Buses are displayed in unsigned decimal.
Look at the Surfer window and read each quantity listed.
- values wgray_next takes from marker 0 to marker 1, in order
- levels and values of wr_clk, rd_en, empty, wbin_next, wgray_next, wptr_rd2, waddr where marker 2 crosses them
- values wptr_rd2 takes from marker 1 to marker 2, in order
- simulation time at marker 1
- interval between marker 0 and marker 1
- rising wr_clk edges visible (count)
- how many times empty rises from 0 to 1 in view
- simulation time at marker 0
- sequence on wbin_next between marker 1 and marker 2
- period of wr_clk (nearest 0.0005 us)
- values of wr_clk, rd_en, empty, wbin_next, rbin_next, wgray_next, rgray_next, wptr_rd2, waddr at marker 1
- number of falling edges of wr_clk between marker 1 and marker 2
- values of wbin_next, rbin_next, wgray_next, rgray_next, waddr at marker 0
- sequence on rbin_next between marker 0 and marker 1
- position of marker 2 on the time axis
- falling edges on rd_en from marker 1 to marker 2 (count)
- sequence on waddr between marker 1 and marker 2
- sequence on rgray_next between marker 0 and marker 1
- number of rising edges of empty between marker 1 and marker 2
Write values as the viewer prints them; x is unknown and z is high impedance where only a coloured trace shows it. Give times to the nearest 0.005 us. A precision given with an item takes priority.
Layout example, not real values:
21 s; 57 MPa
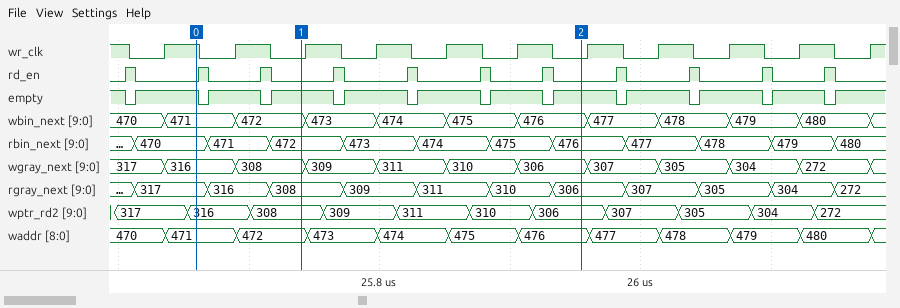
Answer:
316, 308; wr_clk=0, rd_en=0, empty=1, wbin_next=476, wgray_next=306, wptr_rd2=306, waddr=476; 308, 309, 311, 310, 306; 25.74 us; 0.08 us; 11; 11; 25.66 us; 472, 473, 474, 475, 476; 0.054 us; wr_clk=0, rd_en=0, empty=1, wbin_next=472, rbin_next=472, wgray_next=308, rgray_next=308, wptr_rd2=308, waddr=472; 4; wbin_next=471, rbin_next=470, wgray_next=316, rgray_next=317, waddr=471; 470, 471, 472; 25.955 us; 4; 472, 473, 474, 475, 476; 317, 316, 308; 4
